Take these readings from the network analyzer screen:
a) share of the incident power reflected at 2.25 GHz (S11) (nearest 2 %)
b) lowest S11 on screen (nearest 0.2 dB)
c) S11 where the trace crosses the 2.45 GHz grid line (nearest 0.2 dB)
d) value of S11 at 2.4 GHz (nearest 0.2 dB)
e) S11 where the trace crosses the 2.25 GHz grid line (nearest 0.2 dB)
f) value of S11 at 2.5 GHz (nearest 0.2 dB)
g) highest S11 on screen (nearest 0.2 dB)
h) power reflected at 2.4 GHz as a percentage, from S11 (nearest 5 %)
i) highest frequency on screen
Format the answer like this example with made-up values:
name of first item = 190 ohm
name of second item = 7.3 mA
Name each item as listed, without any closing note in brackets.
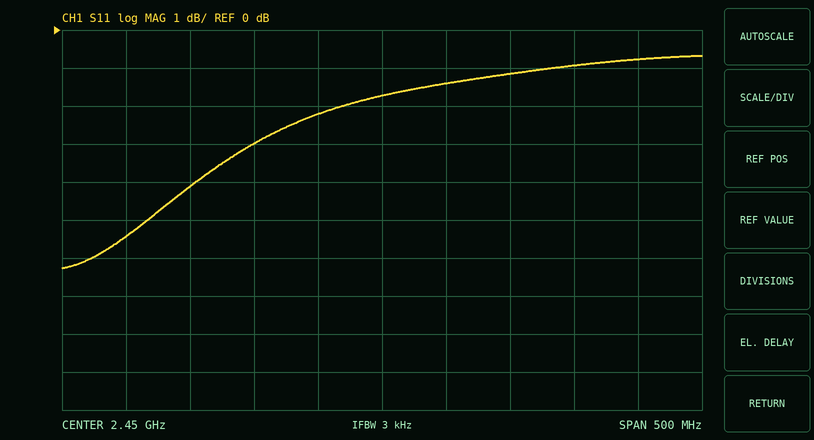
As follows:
share of the incident power reflected at 2.25 GHz (S11) = 28 %
lowest S11 on screen = -6.2 dB
S11 where the trace crosses the 2.45 GHz grid line = -1.8 dB
value of S11 at 2.4 GHz = -2.2 dB
S11 where the trace crosses the 2.25 GHz grid line = -5.4 dB
value of S11 at 2.5 GHz = -1.4 dB
highest S11 on screen = -0.6 dB
power reflected at 2.4 GHz as a percentage, from S11 = 60 %
highest frequency on screen = 2.7 GHz
